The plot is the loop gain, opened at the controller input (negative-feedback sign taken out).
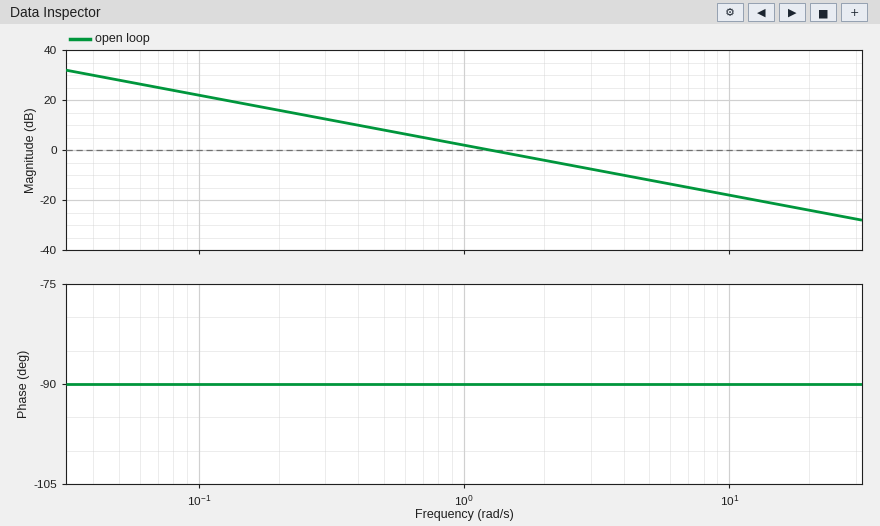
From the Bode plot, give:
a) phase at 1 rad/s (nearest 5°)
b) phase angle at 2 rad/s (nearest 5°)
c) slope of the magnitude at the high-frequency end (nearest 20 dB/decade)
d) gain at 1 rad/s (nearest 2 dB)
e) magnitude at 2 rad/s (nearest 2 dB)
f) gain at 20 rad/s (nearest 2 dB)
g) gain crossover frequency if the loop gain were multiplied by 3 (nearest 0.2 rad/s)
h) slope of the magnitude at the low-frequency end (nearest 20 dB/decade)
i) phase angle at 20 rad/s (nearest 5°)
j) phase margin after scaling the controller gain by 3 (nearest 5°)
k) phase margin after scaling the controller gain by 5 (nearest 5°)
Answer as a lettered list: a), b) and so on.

a) -90°
b) -90°
c) -20 dB/decade
d) 2 dB
e) -4 dB
f) -24 dB
g) 3.8 rad/s
h) -20 dB/decade
i) -90°
j) 90°
k) 90°
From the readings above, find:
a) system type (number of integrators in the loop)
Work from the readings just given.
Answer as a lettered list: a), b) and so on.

a) 1
